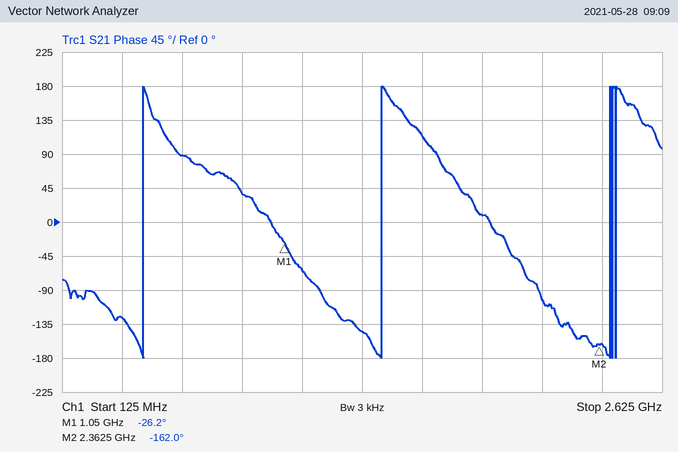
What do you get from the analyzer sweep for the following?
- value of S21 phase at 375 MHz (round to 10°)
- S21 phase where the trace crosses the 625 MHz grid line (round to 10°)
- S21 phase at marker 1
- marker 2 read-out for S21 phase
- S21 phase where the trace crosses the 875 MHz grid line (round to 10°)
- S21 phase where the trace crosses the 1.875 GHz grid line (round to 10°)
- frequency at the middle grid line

-130°
90°
-26.2°
-162.0°
40°
10°
1.375 GHz
